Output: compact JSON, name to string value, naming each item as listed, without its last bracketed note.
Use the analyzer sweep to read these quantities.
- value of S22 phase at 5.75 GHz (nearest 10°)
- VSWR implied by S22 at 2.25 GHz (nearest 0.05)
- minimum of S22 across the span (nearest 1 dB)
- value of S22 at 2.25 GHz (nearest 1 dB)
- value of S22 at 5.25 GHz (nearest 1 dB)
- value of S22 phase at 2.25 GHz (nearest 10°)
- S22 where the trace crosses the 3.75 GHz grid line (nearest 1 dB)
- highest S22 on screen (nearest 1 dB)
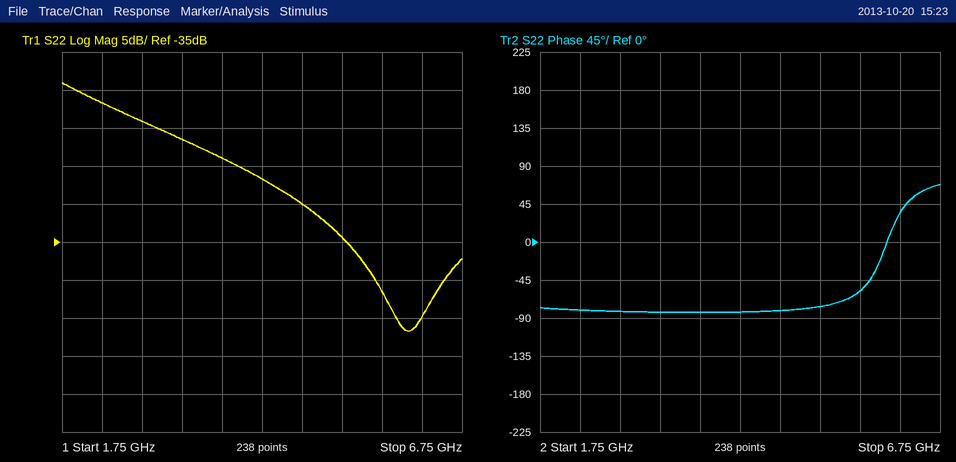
{"value of S22 phase at 5.75 GHz": "-60°", "VSWR implied by S22 at 2.25 GHz": "1.35", "minimum of S22 across the span": "-47 dB", "value of S22 at 2.25 GHz": "-17 dB", "value of S22 at 5.25 GHz": "-34 dB", "value of S22 phase at 2.25 GHz": "-80°", "S22 where the trace crosses the 3.75 GHz grid line": "-24 dB", "highest S22 on screen": "-14 dB"}
